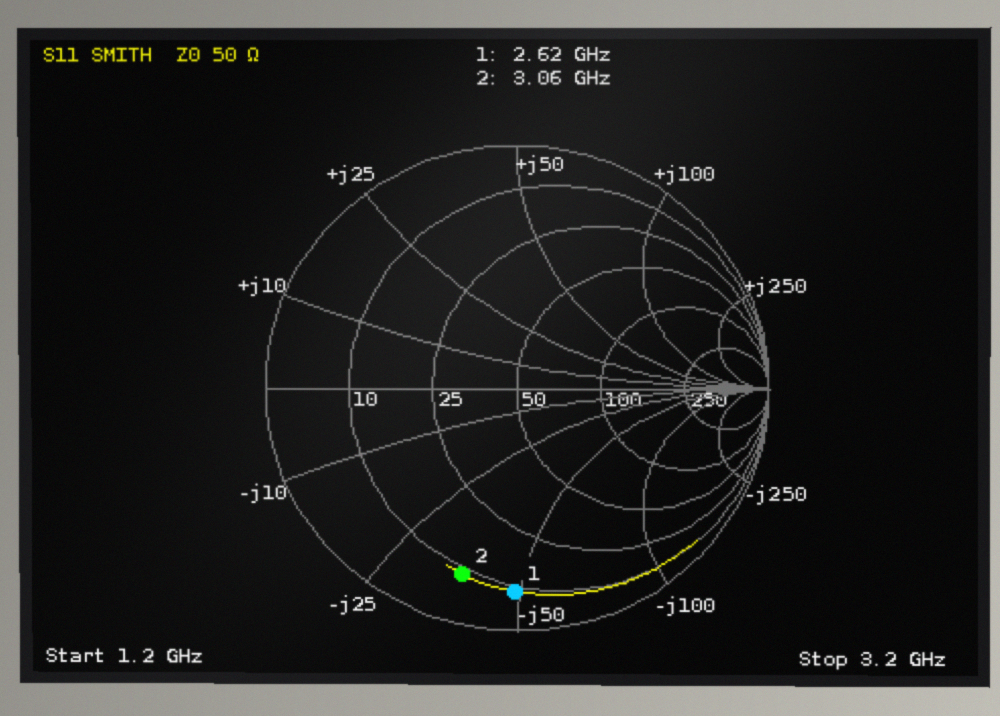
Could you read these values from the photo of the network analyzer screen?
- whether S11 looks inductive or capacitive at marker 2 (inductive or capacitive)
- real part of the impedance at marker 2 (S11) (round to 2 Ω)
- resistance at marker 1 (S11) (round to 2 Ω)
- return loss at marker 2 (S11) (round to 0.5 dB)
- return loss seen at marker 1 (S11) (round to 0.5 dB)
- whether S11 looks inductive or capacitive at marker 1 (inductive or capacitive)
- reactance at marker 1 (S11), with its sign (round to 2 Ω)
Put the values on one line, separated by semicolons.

capacitive; 8 Ω; 8 Ω; 2.0 dB; 1.5 dB; capacitive; -48 Ω
